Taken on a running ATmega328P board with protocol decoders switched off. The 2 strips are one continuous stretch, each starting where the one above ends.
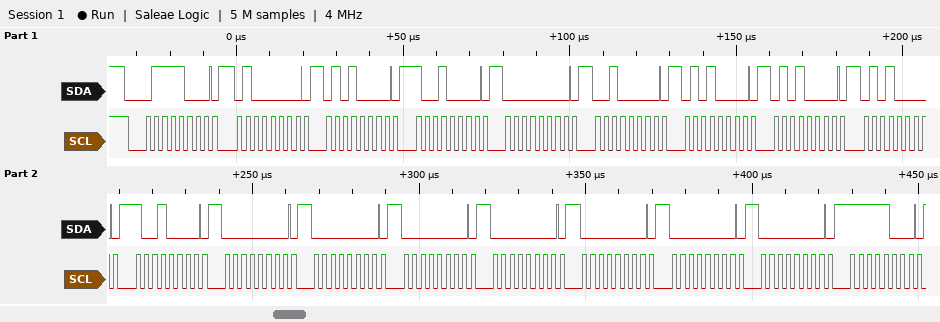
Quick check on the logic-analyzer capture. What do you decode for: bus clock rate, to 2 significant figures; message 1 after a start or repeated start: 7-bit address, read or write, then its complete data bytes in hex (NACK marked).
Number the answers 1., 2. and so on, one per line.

1. 400 kHz
2. 0x3C write: 40 50 90 00 20 50 50 50 90 00 00 00 00 00 00 00 F8
